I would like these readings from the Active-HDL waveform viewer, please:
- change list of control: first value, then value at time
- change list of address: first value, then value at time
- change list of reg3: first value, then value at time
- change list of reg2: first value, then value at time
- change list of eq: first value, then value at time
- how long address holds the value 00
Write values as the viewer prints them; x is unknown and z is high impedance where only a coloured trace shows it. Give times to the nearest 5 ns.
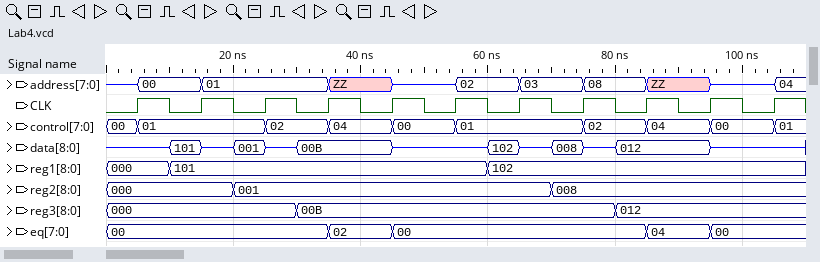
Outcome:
00, 01 at 5 ns, 02 at 25 ns, 04 at 35 ns, 00 at 45 ns, 01 at 55 ns, 02 at 75 ns, 04 at 85 ns, 00 at 95 ns, 01 at 105 ns
z, 00 at 5 ns, 01 at 15 ns, ZZ at 35 ns, z at 45 ns, 02 at 55 ns, 03 at 65 ns, 08 at 75 ns, ZZ at 85 ns, z at 95 ns, 04 at 105 ns
000, 00B at 30 ns, 012 at 80 ns
000, 001 at 20 ns, 008 at 70 ns
00, 02 at 35 ns, 00 at 45 ns, 04 at 85 ns, 00 at 95 ns
10 ns
